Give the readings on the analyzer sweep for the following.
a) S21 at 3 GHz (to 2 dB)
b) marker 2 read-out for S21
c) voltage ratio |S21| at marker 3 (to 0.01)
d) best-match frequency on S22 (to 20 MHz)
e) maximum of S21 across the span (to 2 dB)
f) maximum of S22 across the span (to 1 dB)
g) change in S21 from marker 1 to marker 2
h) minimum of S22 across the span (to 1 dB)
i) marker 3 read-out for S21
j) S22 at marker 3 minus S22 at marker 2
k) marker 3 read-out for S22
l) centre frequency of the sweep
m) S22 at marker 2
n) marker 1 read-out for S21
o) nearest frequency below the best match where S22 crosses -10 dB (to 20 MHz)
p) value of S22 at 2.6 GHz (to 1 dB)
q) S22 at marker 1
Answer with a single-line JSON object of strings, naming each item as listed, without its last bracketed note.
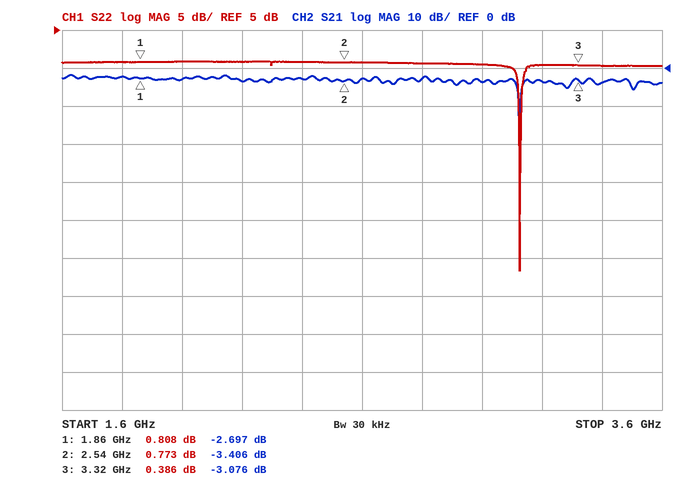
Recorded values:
{"S21 at 3 GHz": "-4 dB", "marker 2 read-out for S21": "-3.406 dB", "voltage ratio |S21| at marker 3": "0.70", "best-match frequency on S22": "3.12 GHz", "maximum of S21 across the span": "-2 dB", "maximum of S22 across the span": "1 dB", "change in S21 from marker 1 to marker 2": "-0.709 dB", "minimum of S22 across the span": "-27 dB", "marker 3 read-out for S21": "-3.076 dB", "S22 at marker 3 minus S22 at marker 2": "-0.387 dB", "marker 3 read-out for S22": "0.386 dB", "centre frequency of the sweep": "2.6 GHz", "S22 at marker 2": "0.773 dB", "marker 1 read-out for S21": "-2.697 dB", "nearest frequency below the best match where S22 crosses -10 dB": "3.12 GHz", "value of S22 at 2.6 GHz": "1 dB", "S22 at marker 1": "0.808 dB"}
